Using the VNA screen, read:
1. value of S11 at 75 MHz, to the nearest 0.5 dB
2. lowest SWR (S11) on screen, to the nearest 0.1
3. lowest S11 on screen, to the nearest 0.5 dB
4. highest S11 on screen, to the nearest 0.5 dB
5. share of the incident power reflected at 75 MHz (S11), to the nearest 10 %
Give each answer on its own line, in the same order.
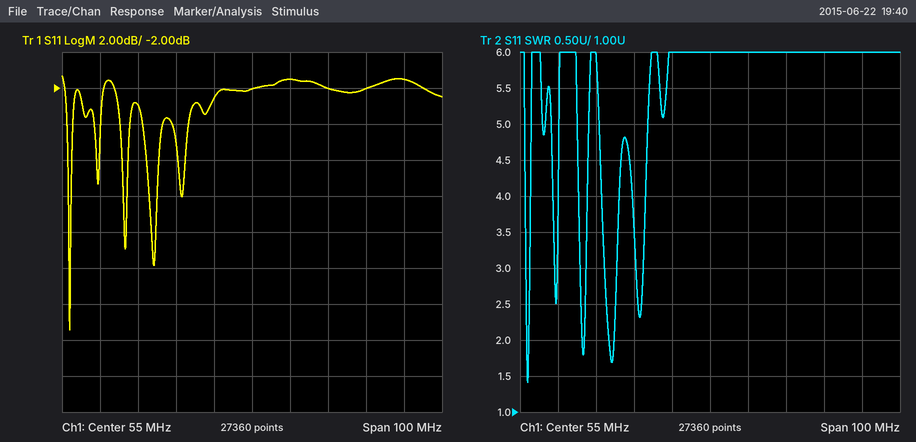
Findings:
-2.0 dB
1.4
-15.5 dB
-1.5 dB
60 %
